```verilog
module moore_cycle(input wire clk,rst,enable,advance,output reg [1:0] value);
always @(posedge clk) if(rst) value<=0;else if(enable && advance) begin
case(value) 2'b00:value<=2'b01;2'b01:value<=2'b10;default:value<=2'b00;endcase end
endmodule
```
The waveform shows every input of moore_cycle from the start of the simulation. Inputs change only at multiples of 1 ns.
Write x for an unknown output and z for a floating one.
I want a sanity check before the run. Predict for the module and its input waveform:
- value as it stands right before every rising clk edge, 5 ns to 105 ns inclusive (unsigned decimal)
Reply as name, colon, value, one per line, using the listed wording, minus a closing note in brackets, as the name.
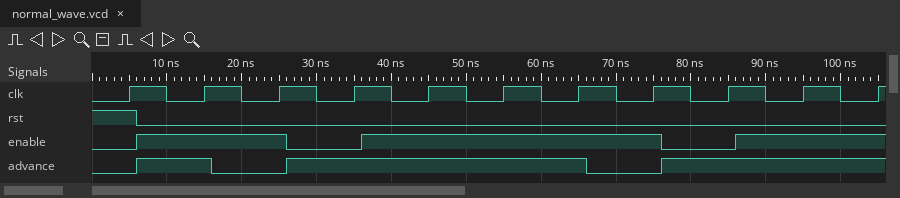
value as it stands right before every rising clk edge, 5 ns to 105 ns inclusive: x, 0, 1, 1, 1, 2, 0, 1, 1, 1, 2
